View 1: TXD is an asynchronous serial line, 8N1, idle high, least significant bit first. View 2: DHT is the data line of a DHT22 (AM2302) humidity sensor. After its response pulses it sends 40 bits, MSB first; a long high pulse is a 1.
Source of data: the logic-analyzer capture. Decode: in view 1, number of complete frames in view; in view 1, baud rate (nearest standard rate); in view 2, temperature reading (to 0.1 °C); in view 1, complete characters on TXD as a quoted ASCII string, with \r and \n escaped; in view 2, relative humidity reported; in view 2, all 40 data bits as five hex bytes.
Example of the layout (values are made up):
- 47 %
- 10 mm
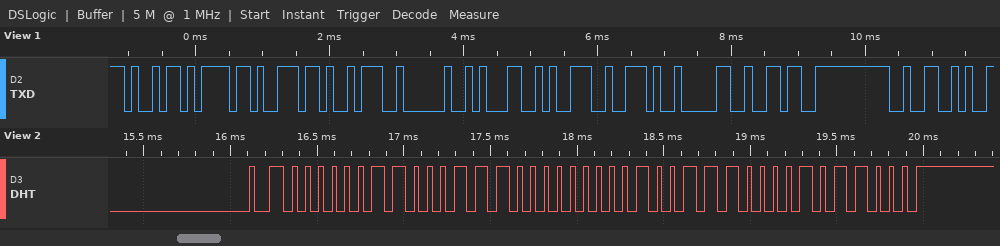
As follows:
- 11
- 9600 baud
- 31.2 °C
- "ion: 19.062"
- 79.6 %
- 03 1C 01 38 58
